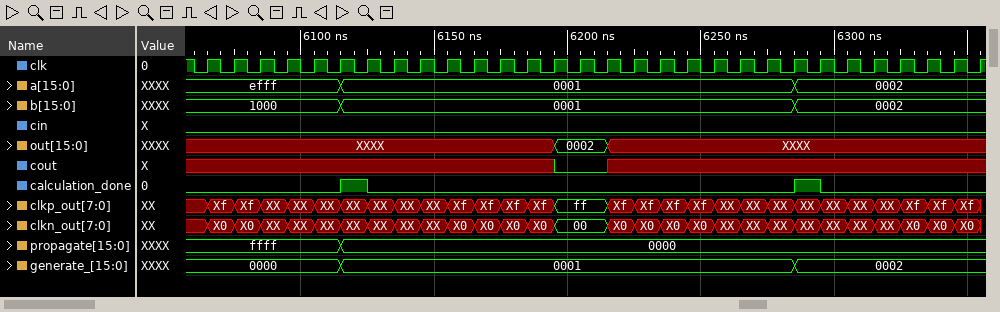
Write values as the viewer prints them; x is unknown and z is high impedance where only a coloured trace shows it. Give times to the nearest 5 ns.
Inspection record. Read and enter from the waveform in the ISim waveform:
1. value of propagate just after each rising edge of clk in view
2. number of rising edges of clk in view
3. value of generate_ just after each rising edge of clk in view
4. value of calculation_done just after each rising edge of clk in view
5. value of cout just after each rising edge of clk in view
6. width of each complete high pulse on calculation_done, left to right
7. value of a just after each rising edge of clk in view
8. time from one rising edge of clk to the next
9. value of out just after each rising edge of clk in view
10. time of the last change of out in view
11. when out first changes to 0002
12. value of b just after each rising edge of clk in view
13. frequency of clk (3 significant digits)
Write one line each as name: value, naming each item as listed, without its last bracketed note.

value of propagate just after each rising edge of clk in view: ffff, ffff, ffff, ffff, ffff, 0000, 0000, 0000, 0000, 0000, 0000, 0000, 0000, 0000, 0000, 0000, 0000, 0000, 0000, 0000, 0000, 0000, 0000, 0000, 0000, 0000, 0000, 0000, 0000, 0000
number of rising edges of clk in view: 30
value of generate_ just after each rising edge of clk in view: 0000, 0000, 0000, 0000, 0000, 0001, 0001, 0001, 0001, 0001, 0001, 0001, 0001, 0001, 0001, 0001, 0001, 0001, 0001, 0001, 0001, 0001, 0002, 0002, 0002, 0002, 0002, 0002, 0002, 0002
value of calculation_done just after each rising edge of clk in view: 0 0 0 0 0 1 0 0 0 0 0 0 0 0 0 0 0 0 0 0 0 0 1 0 0 0 0 0 0 0
value of cout just after each rising edge of clk in view: x x x x x x x x x x x x x 0 0 x x x x x x x x x x x x x x x
width of each complete high pulse on calculation_done, left to right: 10 ns, 10 ns
value of a just after each rising edge of clk in view: efff, efff, efff, efff, efff, 0001, 0001, 0001, 0001, 0001, 0001, 0001, 0001, 0001, 0001, 0001, 0001, 0001, 0001, 0001, 0001, 0001, 0002, 0002, 0002, 0002, 0002, 0002, 0002, 0002
time from one rising edge of clk to the next: 10 ns
value of out just after each rising edge of clk in view: XXXX, XXXX, XXXX, XXXX, XXXX, XXXX, XXXX, XXXX, XXXX, XXXX, XXXX, XXXX, XXXX, 0002, 0002, XXXX, XXXX, XXXX, XXXX, XXXX, XXXX, XXXX, XXXX, XXXX, XXXX, XXXX, XXXX, XXXX, XXXX, XXXX
time of the last change of out in view: 6215 ns
when out first changes to 0002: 6195 ns
value of b just after each rising edge of clk in view: 1000, 1000, 1000, 1000, 1000, 0001, 0001, 0001, 0001, 0001, 0001, 0001, 0001, 0001, 0001, 0001, 0001, 0001, 0001, 0001, 0001, 0001, 0002, 0002, 0002, 0002, 0002, 0002, 0002, 0002
frequency of clk: 100 MHz
